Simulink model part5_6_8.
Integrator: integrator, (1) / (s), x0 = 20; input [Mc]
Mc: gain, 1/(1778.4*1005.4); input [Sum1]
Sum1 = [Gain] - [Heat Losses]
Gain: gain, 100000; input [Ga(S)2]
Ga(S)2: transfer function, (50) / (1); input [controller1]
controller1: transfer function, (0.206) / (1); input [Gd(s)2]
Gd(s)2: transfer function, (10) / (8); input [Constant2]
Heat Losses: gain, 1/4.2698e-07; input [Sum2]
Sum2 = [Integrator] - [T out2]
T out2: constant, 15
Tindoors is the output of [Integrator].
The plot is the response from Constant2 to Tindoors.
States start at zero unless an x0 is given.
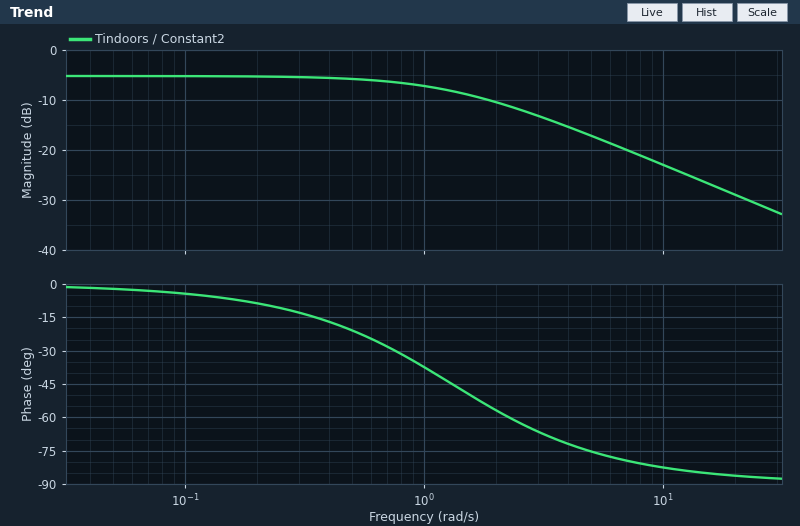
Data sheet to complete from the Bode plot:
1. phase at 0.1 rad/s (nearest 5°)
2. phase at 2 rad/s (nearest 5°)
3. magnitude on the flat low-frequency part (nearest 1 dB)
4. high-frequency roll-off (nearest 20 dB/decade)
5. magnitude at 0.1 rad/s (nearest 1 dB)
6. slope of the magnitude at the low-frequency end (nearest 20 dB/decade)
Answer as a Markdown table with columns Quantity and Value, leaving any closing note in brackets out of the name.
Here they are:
| Quantity | Value |
|---|---|
| phase at 0.1 rad/s | -5° |
| phase at 2 rad/s | -55° |
| magnitude on the flat low-frequency part | -5 dB |
| high-frequency roll-off | -20 dB/decade |
| magnitude at 0.1 rad/s | -5 dB |
| slope of the magnitude at the low-frequency end | 0 dB/decade |
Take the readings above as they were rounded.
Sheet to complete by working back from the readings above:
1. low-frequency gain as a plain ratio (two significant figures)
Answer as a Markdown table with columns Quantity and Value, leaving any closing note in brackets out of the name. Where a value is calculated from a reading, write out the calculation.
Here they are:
| Quantity | Value |
|---|---|
| low-frequency gain as a plain ratio | 10^(-5 / 20) = 0.56 |
